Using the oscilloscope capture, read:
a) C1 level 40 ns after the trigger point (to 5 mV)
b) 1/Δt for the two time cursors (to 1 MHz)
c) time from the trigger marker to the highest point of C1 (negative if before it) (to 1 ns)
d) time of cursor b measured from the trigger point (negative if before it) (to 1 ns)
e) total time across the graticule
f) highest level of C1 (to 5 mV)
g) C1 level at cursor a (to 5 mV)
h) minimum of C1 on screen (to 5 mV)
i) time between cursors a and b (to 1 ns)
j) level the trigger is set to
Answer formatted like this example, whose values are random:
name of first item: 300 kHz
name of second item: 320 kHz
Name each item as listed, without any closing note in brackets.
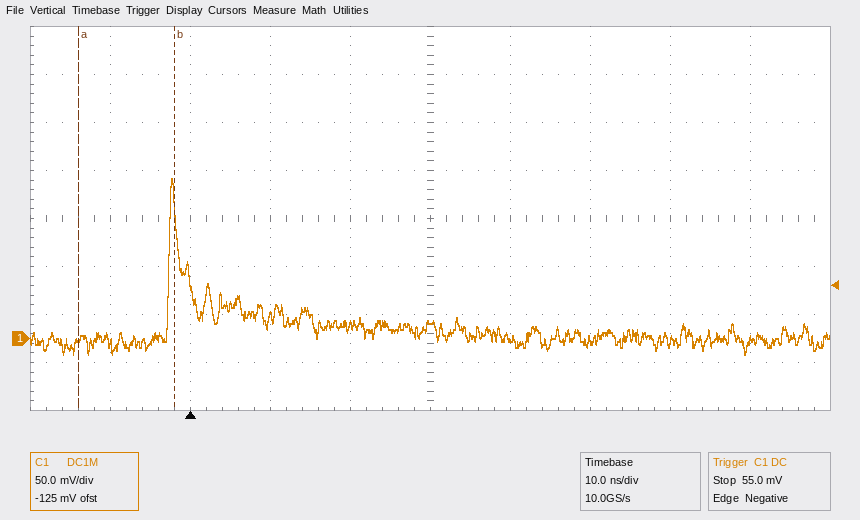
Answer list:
C1 level 40 ns after the trigger point: 0 mV
1/Δt for the two time cursors: 83 MHz
time from the trigger marker to the highest point of C1 (negative if before it): -2 ns
time of cursor b measured from the trigger point (negative if before it): -2 ns
total time across the graticule: 100 ns
highest level of C1: 165 mV
C1 level at cursor a: 0 mV
minimum of C1 on screen: -15 mV
time between cursors a and b: 12 ns
level the trigger is set to: 55.0 mV
